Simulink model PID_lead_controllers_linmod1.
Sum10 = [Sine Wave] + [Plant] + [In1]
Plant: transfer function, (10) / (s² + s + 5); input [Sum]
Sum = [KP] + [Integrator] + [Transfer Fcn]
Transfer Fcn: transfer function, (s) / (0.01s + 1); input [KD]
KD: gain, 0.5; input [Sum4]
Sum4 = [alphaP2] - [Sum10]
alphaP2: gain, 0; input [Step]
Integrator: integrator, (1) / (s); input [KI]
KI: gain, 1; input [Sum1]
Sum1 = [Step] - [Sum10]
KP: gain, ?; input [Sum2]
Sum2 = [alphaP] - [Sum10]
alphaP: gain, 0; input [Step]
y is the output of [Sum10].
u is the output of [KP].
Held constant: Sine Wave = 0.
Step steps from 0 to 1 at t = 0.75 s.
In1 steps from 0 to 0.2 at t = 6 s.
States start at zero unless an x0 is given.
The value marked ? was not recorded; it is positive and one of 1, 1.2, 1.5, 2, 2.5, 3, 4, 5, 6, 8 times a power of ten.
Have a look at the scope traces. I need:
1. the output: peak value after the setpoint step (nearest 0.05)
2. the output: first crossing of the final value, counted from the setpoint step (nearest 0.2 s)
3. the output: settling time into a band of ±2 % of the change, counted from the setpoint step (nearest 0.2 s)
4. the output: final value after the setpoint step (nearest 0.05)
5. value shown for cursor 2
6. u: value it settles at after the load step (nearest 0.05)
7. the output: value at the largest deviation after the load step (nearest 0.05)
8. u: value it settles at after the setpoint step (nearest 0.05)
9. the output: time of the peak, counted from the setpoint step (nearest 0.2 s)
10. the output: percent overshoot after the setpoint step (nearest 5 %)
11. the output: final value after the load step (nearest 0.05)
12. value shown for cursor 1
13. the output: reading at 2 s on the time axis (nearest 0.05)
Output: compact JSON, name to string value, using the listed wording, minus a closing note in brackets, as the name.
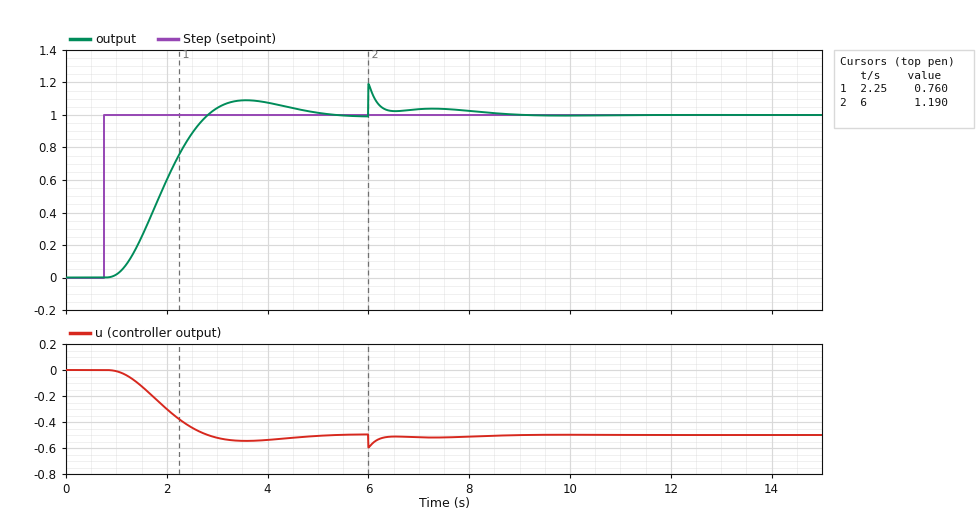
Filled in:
{"the output: peak value after the setpoint step": "1.10", "the output: first crossing of the final value, counted from the setpoint step": "2.0 s", "the output: settling time into a band of ±2 % of the change, counted from the setpoint step": "4.2 s", "the output: final value after the setpoint step": "1.00", "value shown for cursor 2": "1.190", "u: value it settles at after the load step": "-0.50", "the output: value at the largest deviation after the load step": "1.20", "u: value it settles at after the setpoint step": "-0.50", "the output: time of the peak, counted from the setpoint step": "2.8 s", "the output: percent overshoot after the setpoint step": "10 %", "the output: final value after the load step": "1.00", "value shown for cursor 1": "0.760", "the output: reading at 2 s on the time axis": "0.60"}
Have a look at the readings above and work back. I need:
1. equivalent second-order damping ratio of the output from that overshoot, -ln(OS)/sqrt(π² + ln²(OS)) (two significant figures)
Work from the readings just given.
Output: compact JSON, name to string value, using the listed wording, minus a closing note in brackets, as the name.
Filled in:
{"equivalent second-order damping ratio of the output from that overshoot, -ln(OS)/sqrt(π² + ln²(OS))": "0.59"}
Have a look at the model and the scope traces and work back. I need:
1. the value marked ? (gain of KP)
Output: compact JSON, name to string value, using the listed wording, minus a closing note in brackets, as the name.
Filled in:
{"the value marked ?": "0.5"}
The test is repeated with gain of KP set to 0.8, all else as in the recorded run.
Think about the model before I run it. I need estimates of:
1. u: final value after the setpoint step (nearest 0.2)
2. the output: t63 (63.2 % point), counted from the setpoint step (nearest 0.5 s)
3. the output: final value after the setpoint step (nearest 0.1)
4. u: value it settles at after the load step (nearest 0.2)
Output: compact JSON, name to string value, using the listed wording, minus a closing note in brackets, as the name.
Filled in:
{"u: final value after the setpoint step": "-0.8", "the output: t63 (63.2 % point), counted from the setpoint step": "1.5 s", "the output: final value after the setpoint step": "1.0", "u: value it settles at after the load step": "-0.8"}
